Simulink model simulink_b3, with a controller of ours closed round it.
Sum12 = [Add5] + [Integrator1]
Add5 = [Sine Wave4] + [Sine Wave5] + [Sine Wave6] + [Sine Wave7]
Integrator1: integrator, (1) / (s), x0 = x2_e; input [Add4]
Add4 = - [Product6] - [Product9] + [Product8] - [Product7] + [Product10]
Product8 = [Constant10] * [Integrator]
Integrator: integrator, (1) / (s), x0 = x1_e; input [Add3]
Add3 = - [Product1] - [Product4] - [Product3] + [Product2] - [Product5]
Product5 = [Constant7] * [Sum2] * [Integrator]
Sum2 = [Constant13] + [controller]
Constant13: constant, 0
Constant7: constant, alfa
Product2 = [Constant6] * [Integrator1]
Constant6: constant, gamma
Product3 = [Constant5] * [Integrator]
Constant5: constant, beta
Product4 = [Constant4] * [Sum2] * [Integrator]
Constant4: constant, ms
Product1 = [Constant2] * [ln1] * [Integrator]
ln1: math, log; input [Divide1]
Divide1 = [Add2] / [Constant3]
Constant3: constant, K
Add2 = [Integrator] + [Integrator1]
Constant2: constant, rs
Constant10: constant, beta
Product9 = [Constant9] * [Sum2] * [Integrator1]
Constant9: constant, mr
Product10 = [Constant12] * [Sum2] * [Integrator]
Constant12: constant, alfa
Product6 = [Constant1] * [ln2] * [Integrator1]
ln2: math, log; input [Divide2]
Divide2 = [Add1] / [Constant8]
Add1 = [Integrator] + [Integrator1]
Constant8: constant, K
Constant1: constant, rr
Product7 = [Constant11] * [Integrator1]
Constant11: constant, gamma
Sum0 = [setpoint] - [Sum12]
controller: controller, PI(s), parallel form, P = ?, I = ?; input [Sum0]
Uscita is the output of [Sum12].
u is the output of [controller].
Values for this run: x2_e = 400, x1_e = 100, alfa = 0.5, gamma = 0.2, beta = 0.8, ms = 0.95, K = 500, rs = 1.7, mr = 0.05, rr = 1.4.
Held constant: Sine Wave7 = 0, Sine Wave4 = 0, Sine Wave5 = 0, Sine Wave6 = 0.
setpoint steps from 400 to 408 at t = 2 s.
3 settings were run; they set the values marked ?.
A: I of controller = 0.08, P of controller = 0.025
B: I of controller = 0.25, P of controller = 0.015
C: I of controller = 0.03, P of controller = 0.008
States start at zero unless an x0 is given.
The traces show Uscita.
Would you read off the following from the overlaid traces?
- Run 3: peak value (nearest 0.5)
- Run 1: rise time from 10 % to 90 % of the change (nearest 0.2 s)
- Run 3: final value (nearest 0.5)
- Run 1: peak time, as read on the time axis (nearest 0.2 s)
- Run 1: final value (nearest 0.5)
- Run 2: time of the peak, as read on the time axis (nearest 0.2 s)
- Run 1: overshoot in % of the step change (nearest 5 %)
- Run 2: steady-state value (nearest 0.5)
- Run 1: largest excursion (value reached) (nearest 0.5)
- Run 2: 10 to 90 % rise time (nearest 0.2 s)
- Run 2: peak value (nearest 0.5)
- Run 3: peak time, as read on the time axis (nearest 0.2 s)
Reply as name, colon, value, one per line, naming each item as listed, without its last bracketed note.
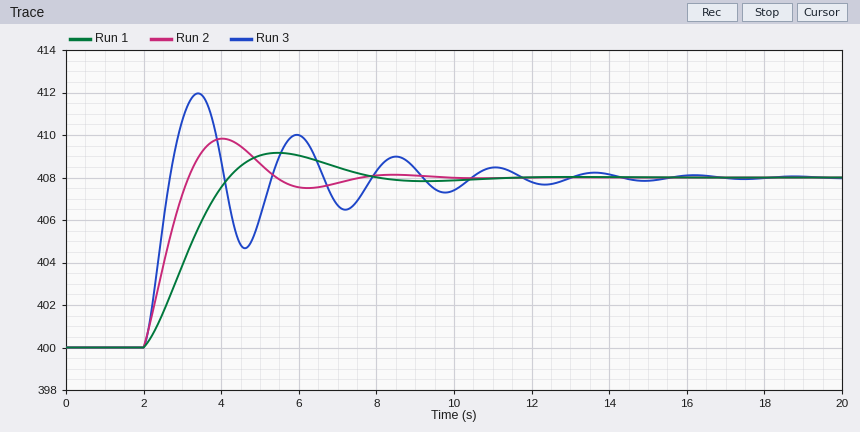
Run 3: peak value: 412.0
Run 1: rise time from 10 % to 90 % of the change: 1.6 s
Run 3: final value: 408.0
Run 1: peak time, as read on the time axis: 5.4 s
Run 1: final value: 408.0
Run 2: time of the peak, as read on the time axis: 4.0 s
Run 1: overshoot in % of the step change: 15 %
Run 2: steady-state value: 408.0
Run 1: largest excursion (value reached): 409.0
Run 2: 10 to 90 % rise time: 0.8 s
Run 2: peak value: 410.0
Run 3: peak time, as read on the time axis: 3.4 s
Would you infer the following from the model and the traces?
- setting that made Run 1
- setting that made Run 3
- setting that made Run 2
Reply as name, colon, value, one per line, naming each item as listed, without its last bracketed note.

setting that made Run 1: C
setting that made Run 3: B
setting that made Run 2: A
